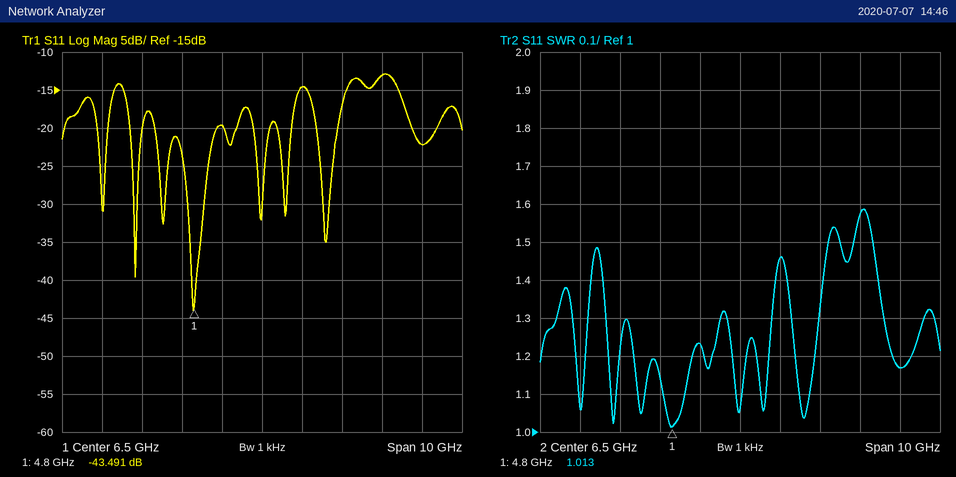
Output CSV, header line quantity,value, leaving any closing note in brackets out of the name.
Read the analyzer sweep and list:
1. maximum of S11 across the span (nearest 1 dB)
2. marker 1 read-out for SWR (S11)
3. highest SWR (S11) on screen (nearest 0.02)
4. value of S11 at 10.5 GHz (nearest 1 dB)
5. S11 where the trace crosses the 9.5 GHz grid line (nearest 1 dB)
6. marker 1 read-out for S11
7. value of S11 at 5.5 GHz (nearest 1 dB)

quantity,value
maximum of S11 across the span,-13 dB
marker 1 read-out for SWR,1.013
highest SWR (S11) on screen,1.58
value of S11 at 10.5 GHz,-22 dB
S11 where the trace crosses the 9.5 GHz grid line,-13 dB
marker 1 read-out for S11,-43.491 dB
value of S11 at 5.5 GHz,-20 dB
